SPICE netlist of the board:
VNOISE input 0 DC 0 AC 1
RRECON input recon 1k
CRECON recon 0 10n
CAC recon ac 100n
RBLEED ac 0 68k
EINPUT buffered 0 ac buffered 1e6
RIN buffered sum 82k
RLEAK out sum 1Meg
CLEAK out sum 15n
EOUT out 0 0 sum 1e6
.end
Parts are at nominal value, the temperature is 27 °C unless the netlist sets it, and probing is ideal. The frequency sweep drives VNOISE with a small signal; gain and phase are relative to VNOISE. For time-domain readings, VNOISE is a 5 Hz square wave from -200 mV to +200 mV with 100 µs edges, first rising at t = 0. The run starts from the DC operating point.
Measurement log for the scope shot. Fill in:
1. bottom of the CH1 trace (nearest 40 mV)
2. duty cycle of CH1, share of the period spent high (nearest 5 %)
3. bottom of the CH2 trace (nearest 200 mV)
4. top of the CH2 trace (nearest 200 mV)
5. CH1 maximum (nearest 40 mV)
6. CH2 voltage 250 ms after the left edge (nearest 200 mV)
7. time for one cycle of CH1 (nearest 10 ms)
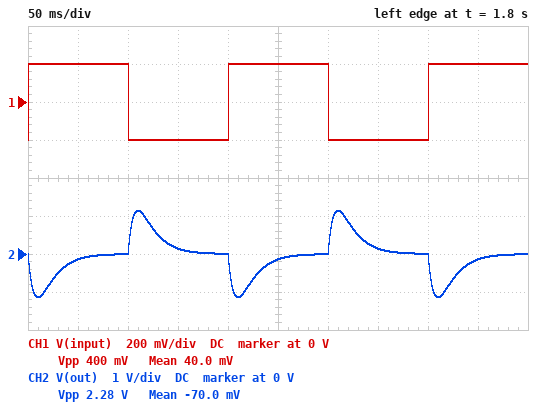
-200 mV
50 %
-1.2 V
1.2 V
200 mV
-200 mV
200 ms
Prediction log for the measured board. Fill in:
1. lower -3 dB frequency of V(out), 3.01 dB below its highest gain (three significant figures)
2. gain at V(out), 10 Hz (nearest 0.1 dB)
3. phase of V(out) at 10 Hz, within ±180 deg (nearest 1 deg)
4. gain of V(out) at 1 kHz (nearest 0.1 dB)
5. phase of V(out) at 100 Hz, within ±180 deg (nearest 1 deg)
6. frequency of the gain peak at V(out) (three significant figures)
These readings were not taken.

6.15 Hz
10.8 dB
-157 deg
-17.9 dB
109 deg
15.6 Hz
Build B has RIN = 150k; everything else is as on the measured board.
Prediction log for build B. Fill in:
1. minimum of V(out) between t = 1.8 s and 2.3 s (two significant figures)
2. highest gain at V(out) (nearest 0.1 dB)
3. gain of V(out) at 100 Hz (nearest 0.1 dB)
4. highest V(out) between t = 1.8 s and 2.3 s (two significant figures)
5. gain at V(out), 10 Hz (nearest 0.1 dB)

-620 mV
6.3 dB
-3.4 dB
620 mV
5.6 dB
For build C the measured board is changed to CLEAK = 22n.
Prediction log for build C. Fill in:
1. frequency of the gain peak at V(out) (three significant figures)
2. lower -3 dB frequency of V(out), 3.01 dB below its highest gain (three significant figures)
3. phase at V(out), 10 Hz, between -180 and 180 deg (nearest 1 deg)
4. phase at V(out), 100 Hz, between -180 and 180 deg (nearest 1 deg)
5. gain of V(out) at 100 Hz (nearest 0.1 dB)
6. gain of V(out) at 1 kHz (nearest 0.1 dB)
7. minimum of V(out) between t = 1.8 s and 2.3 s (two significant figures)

12.9 Hz
4.76 Hz
-168 deg
107 deg
-1.5 dB
-21.2 dB
-870 mV
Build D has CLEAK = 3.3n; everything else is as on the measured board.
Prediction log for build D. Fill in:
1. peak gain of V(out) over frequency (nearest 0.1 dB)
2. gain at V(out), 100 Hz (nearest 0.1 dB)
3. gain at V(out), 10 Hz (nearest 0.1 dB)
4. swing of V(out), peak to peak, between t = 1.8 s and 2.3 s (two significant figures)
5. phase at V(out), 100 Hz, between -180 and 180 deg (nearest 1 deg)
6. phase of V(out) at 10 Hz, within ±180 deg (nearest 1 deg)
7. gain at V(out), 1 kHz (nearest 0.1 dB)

18.2 dB
14.1 dB
13.4 dB
4.9 V
128 deg
-125 deg
-4.8 dB
